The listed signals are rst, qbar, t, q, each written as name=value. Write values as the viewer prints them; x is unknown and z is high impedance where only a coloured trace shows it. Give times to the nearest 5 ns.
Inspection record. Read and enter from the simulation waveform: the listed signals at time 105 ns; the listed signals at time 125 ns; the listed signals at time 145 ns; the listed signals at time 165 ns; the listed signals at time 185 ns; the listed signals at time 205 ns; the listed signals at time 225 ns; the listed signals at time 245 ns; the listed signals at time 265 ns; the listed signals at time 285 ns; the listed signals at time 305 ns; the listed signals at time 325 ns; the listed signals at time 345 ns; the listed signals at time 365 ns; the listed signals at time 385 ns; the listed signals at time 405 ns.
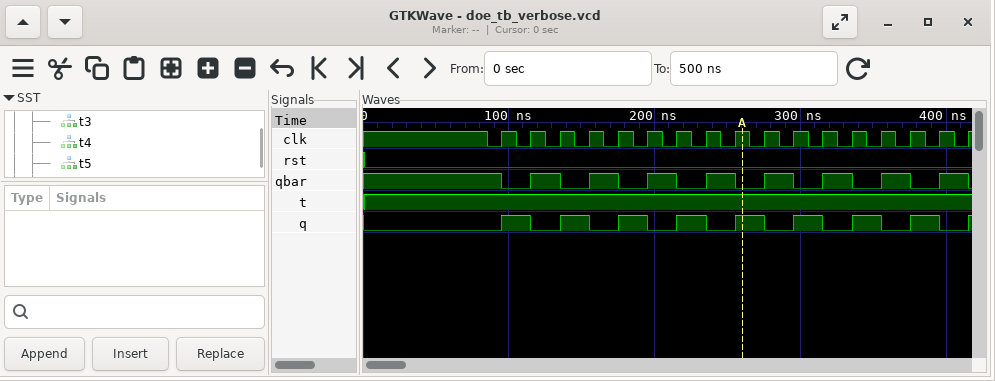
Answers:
rst=0, qbar=0, t=1, q=1
rst=0, qbar=1, t=1, q=0
rst=0, qbar=0, t=1, q=1
rst=0, qbar=1, t=1, q=0
rst=0, qbar=0, t=1, q=1
rst=0, qbar=1, t=1, q=0
rst=0, qbar=0, t=1, q=1
rst=0, qbar=1, t=1, q=0
rst=0, qbar=0, t=1, q=1
rst=0, qbar=1, t=1, q=0
rst=0, qbar=0, t=1, q=1
rst=0, qbar=1, t=1, q=0
rst=0, qbar=0, t=1, q=1
rst=0, qbar=1, t=1, q=0
rst=0, qbar=0, t=1, q=1
rst=0, qbar=1, t=1, q=0
